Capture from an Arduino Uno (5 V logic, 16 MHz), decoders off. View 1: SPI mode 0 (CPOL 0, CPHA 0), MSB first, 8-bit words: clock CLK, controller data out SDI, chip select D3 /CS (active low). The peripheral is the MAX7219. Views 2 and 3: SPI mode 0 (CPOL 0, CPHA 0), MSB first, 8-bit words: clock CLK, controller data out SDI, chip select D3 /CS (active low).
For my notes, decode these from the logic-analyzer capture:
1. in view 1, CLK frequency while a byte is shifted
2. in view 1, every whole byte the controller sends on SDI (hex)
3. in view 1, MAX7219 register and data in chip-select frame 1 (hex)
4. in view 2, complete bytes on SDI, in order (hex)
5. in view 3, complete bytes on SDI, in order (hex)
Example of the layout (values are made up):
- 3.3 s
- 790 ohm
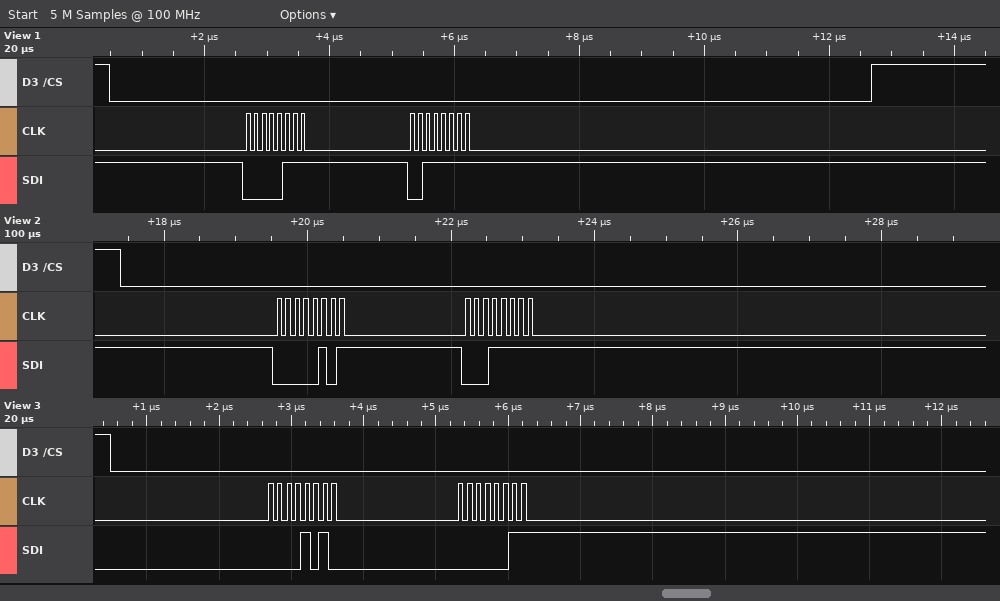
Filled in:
- 8 MHz
- 07 3F
- register 0x7, data 0x3F
- 0x05 0x1F
- 0A 03
